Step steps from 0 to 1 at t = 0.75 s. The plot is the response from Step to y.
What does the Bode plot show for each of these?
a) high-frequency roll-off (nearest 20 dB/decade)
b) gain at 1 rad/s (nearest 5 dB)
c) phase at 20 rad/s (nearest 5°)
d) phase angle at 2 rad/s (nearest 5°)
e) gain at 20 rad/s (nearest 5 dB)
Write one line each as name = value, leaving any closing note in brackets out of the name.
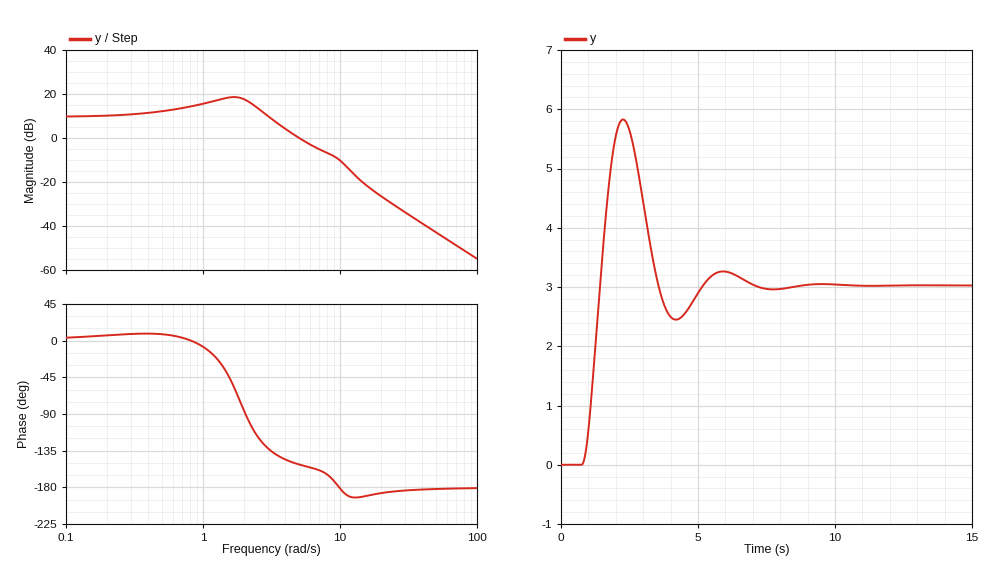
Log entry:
high-frequency roll-off = -40 dB/decade
gain at 1 rad/s = 15 dB
phase at 20 rad/s = -185°
phase angle at 2 rad/s = -85°
gain at 20 rad/s = -25 dB
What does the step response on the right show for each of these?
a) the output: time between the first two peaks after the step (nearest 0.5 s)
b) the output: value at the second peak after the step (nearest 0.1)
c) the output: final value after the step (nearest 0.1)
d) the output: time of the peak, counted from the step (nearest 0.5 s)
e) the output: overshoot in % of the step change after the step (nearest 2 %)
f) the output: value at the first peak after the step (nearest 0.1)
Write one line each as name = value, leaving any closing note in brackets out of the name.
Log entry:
the output: time between the first two peaks after the step = 3.5 s
the output: value at the second peak after the step = 3.3
the output: final value after the step = 3.0
the output: time of the peak, counted from the step = 1.5 s
the output: overshoot in % of the step change after the step = 92 %
the output: value at the first peak after the step = 5.8
